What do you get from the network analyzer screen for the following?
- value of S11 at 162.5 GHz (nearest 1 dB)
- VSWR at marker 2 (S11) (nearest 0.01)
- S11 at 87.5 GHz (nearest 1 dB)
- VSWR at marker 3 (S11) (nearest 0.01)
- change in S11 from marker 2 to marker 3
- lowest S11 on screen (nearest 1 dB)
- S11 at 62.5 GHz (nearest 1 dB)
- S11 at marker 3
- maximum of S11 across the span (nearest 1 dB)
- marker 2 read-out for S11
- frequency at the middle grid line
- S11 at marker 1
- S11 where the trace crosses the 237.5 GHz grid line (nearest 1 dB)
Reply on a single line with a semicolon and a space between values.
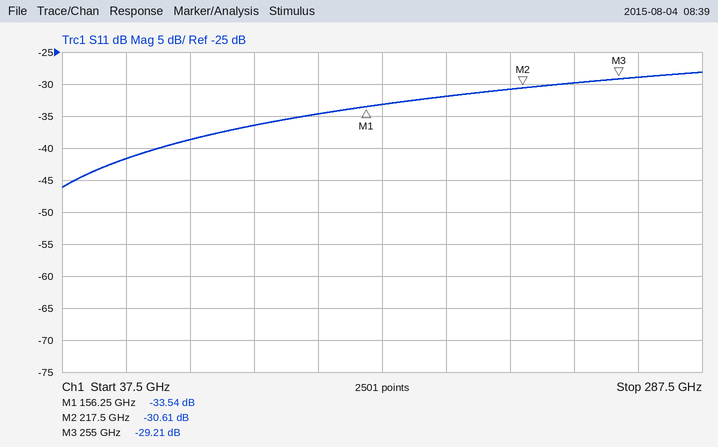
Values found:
-33 dB; 1.06; -39 dB; 1.07; 1.40 dB; -46 dB; -42 dB; -29.21 dB; -28 dB; -30.61 dB; 162.5 GHz; -33.54 dB; -30 dB
